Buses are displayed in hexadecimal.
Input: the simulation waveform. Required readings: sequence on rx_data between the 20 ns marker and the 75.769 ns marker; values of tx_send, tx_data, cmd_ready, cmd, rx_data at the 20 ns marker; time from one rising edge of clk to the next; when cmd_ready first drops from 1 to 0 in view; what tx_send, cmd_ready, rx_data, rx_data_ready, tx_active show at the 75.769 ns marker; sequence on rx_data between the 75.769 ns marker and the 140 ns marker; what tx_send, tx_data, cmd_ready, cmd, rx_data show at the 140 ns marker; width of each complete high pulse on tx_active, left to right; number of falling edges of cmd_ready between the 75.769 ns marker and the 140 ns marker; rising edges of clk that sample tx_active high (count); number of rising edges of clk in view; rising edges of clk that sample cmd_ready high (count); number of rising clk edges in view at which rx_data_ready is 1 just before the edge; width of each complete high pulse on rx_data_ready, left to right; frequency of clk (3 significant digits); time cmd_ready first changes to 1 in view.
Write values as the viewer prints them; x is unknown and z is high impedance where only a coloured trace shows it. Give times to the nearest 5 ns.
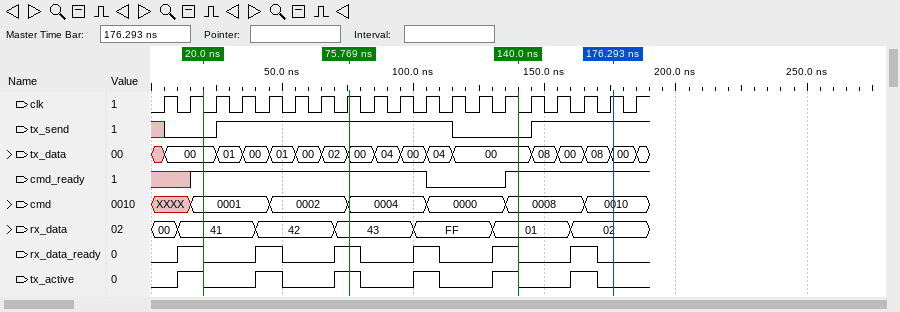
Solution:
41, 42, 43
tx_send=0, tx_data=00, cmd_ready=1, cmd=0001, rx_data=41
10 ns
105 ns
tx_send=1, cmd_ready=1, rx_data=43, rx_data_ready=1, tx_active=1
43, FF, 01
tx_send=0, tx_data=00, cmd_ready=1, cmd=0008, rx_data=01
10 ns, 10 ns, 10 ns, 10 ns, 10 ns, 10 ns
1
6
19
14
6
10 ns, 10 ns, 10 ns, 10 ns, 10 ns, 10 ns
100 MHz
15 ns
